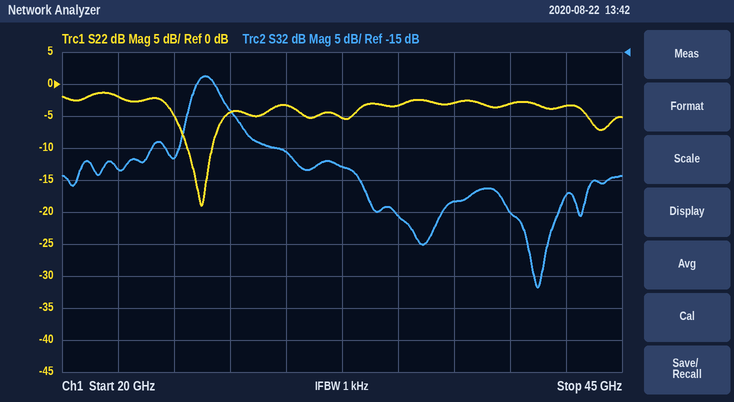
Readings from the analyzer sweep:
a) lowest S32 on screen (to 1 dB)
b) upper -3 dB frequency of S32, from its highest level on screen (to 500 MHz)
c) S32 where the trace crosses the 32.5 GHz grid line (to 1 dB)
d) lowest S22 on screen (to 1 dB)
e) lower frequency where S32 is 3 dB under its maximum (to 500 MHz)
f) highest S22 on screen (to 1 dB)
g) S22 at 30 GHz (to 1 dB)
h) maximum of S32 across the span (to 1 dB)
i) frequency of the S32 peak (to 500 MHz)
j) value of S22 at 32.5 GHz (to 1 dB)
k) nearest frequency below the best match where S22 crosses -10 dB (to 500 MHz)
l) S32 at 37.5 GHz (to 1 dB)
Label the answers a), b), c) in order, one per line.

a) -52 dB
b) 27.0 GHz
c) -33 dB
d) -19 dB
e) 26.0 GHz
f) -1 dB
g) -3 dB
h) -19 dB
i) 26.5 GHz
j) -5 dB
k) 25.5 GHz
l) -38 dB
